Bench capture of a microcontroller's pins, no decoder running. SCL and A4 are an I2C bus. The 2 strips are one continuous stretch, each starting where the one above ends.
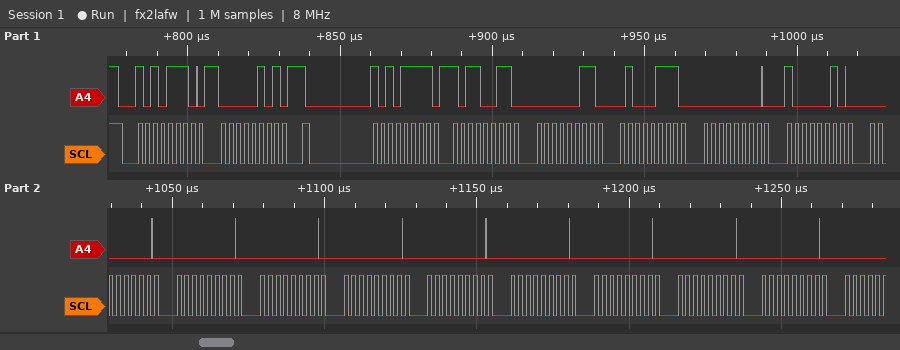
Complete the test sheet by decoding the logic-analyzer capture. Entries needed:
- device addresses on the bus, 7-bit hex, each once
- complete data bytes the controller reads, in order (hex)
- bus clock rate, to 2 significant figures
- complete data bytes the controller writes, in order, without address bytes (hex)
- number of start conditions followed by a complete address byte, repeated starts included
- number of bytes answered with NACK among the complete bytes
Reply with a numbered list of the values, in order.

1. 0x57
2. B3 03 47 00 82 00 00 00 00 00 00 00 00 00
3. 400 kHz
4. 05
5. 2
6. 0
